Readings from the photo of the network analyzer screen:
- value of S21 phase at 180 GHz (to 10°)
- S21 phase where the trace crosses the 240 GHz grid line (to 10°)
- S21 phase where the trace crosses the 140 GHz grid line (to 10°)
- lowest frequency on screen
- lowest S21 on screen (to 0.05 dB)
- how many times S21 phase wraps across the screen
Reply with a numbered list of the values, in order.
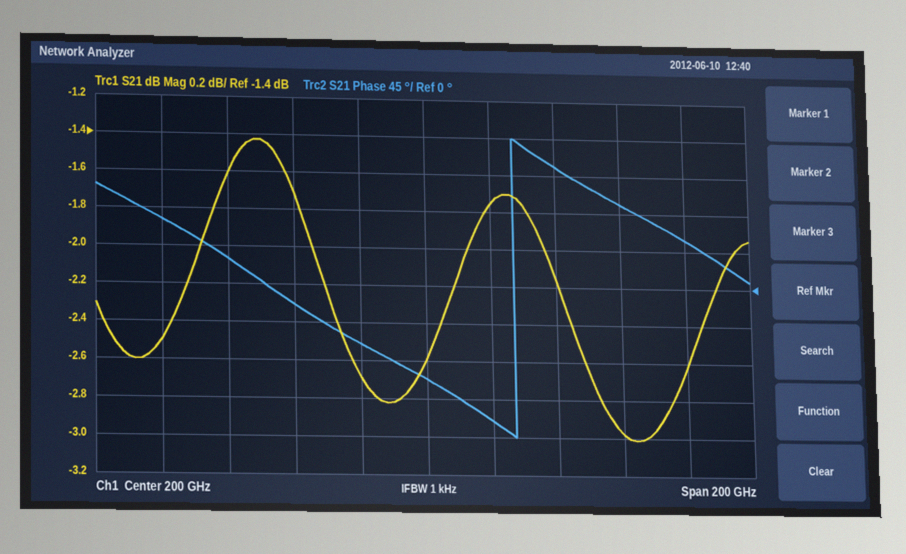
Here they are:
1. -70°
2. 150°
3. 30°
4. 100 GHz
5. -3.00 dB
6. 1
